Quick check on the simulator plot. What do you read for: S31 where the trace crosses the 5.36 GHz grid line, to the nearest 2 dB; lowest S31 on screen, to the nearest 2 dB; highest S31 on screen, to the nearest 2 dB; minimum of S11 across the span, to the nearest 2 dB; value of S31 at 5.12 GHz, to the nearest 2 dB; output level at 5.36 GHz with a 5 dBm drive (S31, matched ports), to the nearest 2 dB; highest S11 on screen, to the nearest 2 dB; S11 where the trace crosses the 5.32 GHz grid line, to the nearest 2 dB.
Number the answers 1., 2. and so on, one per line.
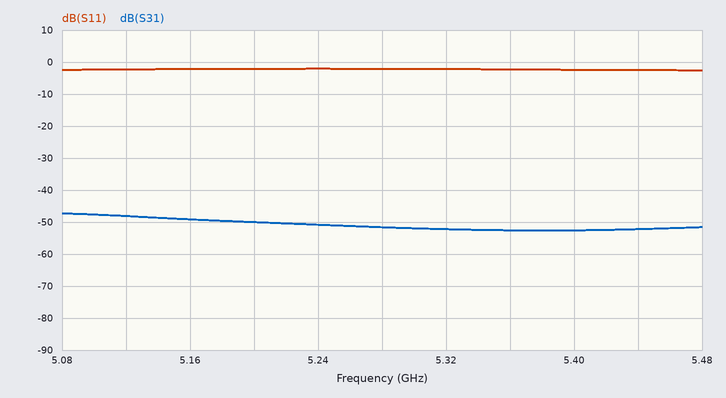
1. -52 dB
2. -52 dB
3. -48 dB
4. -2 dB
5. -48 dB
6. -48 dBm
7. -2 dB
8. -2 dB
